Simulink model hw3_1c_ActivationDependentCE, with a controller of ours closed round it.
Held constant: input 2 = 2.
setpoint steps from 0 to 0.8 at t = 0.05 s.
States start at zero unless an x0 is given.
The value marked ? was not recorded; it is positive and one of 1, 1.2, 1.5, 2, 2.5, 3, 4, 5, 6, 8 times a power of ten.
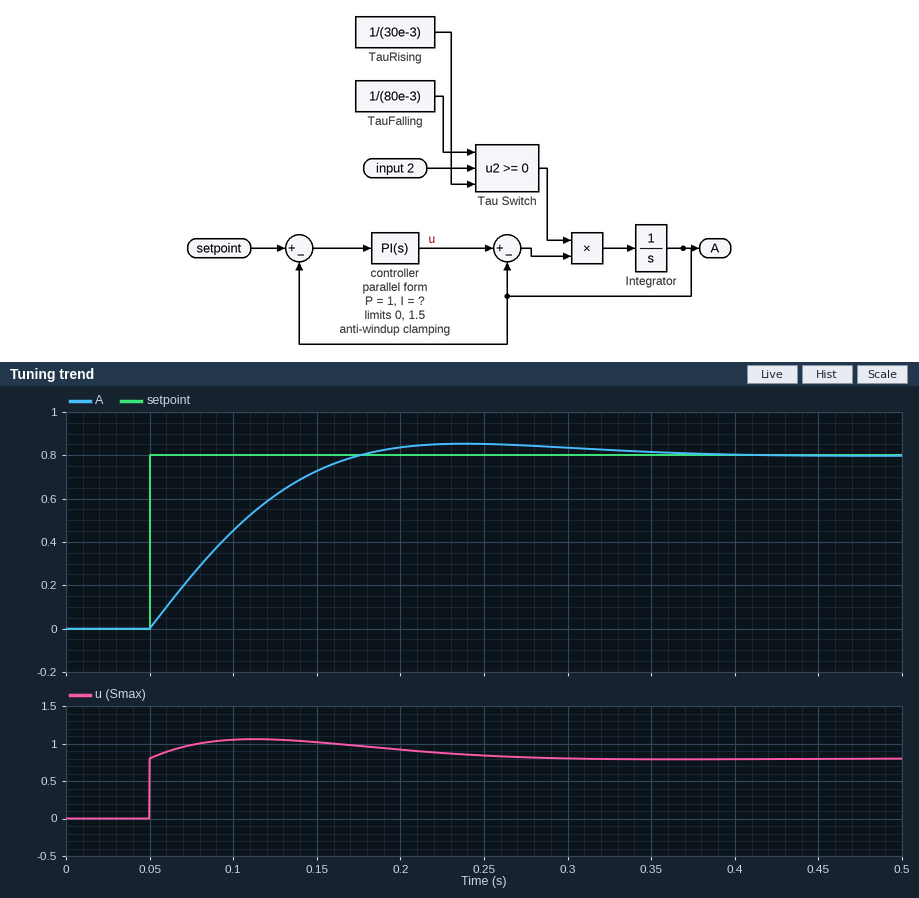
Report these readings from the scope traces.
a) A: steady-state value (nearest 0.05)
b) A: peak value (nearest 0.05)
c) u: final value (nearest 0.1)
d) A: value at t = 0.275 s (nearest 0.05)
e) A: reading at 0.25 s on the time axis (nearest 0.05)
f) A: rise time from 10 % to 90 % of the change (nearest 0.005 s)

0.80
0.85
0.8
0.85
0.85
0.090 s
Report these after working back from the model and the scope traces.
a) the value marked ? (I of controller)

25
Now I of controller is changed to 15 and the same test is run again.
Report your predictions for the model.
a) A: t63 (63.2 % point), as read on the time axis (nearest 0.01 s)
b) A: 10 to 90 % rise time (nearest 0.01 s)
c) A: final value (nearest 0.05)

0.12 s
0.14 s
0.80
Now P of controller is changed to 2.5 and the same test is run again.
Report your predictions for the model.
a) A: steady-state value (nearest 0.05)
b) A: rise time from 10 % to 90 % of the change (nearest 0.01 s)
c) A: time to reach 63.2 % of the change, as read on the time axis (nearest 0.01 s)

0.80
0.11 s
0.09 s
